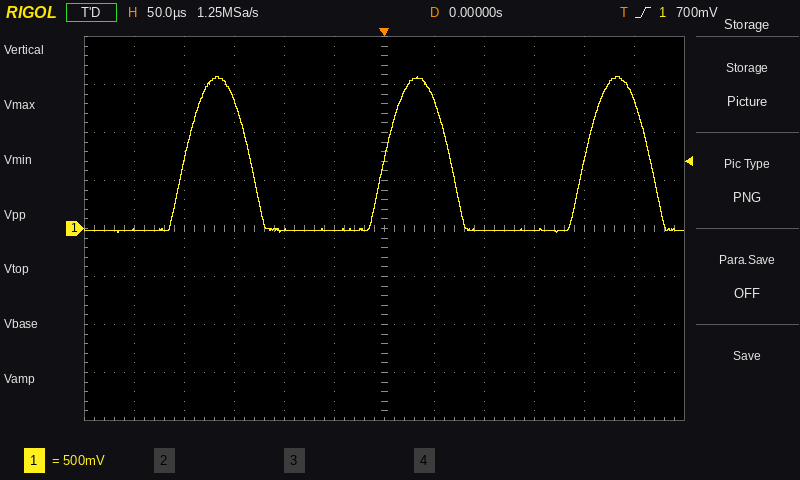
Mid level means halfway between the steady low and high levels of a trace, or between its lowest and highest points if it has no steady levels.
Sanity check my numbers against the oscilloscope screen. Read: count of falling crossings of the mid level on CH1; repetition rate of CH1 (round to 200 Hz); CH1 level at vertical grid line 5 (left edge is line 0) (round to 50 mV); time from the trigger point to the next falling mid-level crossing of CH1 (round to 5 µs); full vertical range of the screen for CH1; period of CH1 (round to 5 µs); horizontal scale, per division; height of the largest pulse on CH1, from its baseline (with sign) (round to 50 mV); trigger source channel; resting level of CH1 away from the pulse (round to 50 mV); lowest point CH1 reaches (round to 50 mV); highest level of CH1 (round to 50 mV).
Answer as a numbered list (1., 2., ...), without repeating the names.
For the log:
1. 3
2. 5.0 kHz
3. 0 mV
4. 65 µs
5. 4 V
6. 200 µs
7. 50 µs
8. +1.60 V
9. CH1
10. 0 mV
11. -50 mV
12. 1.60 V
